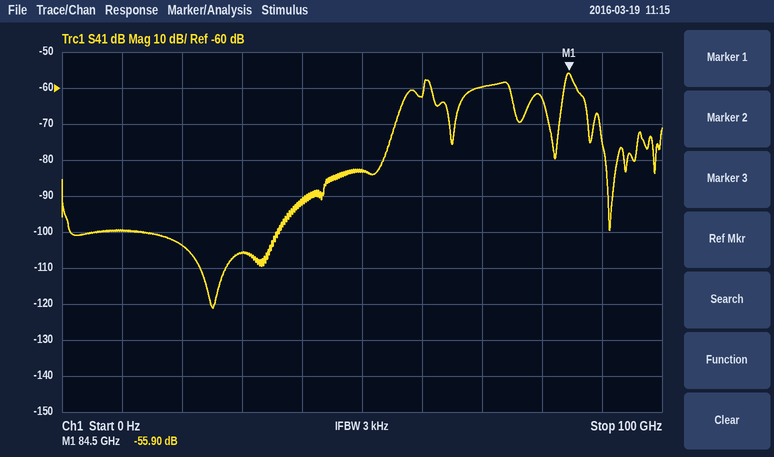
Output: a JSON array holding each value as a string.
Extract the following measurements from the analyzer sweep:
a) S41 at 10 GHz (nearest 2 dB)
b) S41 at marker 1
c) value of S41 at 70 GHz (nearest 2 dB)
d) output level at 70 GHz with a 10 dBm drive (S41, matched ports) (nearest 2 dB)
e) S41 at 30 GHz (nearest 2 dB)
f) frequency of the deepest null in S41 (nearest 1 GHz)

["-100 dB", "-55.90 dB", "-60 dB", "-50 dBm", "-106 dB", "25 GHz"]
